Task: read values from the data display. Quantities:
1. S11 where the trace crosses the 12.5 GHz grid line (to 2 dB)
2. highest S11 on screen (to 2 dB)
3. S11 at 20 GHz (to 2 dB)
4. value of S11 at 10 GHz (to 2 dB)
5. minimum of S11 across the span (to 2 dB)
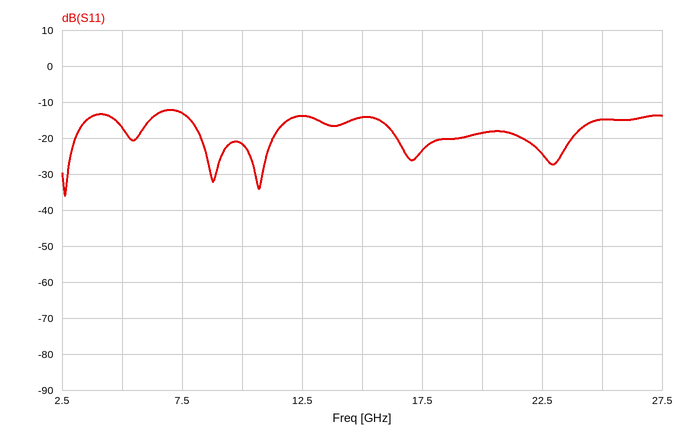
-14 dB
-12 dB
-18 dB
-22 dB
-36 dB
